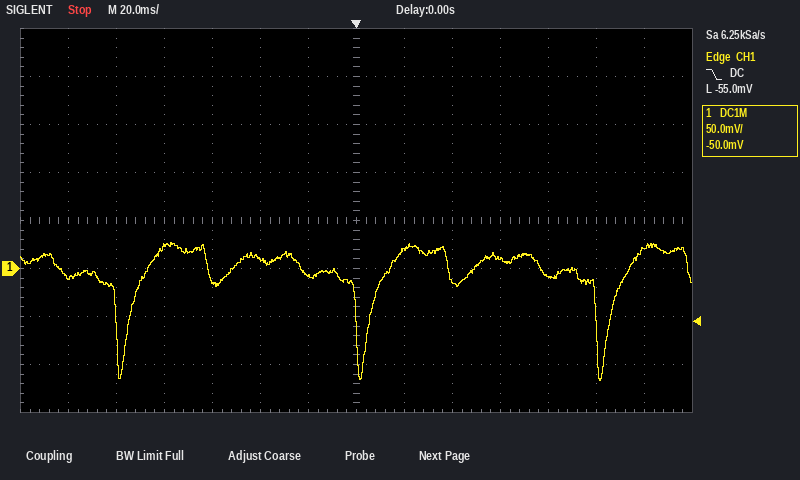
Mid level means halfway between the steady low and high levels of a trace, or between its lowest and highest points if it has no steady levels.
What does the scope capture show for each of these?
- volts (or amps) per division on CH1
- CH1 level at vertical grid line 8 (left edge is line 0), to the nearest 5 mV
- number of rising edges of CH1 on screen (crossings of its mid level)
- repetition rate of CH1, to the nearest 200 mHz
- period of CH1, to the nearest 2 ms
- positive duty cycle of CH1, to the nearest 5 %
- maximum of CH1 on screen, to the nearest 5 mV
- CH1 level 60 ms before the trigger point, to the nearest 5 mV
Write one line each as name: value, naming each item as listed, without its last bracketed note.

volts (or amps) per division on CH1: 50 mV
CH1 level at vertical grid line 8 (left edge is line 0), to the nearest 5 mV: 20 mV
number of rising edges of CH1 on screen: 3
repetition rate of CH1, to the nearest 200 mHz: 10.0 Hz
period of CH1, to the nearest 2 ms: 100 ms
positive duty cycle of CH1, to the nearest 5 %: 95 %
maximum of CH1 on screen, to the nearest 5 mV: 25 mV
CH1 level 60 ms before the trigger point, to the nearest 5 mV: -15 mV
